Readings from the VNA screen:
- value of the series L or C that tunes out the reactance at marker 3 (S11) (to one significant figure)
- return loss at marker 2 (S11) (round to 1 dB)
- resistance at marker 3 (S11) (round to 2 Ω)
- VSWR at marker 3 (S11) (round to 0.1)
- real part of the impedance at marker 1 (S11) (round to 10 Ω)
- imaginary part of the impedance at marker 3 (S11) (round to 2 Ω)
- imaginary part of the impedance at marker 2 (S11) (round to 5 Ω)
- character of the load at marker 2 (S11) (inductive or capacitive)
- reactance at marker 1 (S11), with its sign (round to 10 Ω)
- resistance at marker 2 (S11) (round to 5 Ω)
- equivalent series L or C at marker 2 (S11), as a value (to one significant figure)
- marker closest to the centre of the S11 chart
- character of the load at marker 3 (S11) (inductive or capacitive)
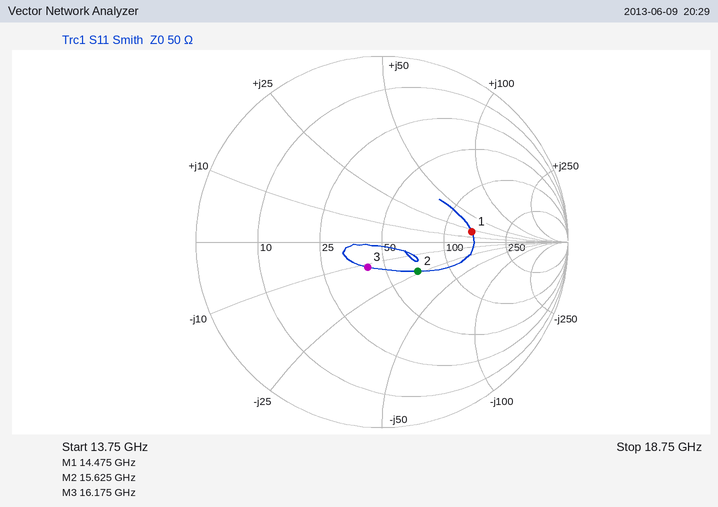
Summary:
100 pH
12 dB
42 Ω
1.4
140 Ω
-12 Ω
-25 Ω
capacitive
+20 Ω
70 Ω
400 fF
marker 3
capacitive
